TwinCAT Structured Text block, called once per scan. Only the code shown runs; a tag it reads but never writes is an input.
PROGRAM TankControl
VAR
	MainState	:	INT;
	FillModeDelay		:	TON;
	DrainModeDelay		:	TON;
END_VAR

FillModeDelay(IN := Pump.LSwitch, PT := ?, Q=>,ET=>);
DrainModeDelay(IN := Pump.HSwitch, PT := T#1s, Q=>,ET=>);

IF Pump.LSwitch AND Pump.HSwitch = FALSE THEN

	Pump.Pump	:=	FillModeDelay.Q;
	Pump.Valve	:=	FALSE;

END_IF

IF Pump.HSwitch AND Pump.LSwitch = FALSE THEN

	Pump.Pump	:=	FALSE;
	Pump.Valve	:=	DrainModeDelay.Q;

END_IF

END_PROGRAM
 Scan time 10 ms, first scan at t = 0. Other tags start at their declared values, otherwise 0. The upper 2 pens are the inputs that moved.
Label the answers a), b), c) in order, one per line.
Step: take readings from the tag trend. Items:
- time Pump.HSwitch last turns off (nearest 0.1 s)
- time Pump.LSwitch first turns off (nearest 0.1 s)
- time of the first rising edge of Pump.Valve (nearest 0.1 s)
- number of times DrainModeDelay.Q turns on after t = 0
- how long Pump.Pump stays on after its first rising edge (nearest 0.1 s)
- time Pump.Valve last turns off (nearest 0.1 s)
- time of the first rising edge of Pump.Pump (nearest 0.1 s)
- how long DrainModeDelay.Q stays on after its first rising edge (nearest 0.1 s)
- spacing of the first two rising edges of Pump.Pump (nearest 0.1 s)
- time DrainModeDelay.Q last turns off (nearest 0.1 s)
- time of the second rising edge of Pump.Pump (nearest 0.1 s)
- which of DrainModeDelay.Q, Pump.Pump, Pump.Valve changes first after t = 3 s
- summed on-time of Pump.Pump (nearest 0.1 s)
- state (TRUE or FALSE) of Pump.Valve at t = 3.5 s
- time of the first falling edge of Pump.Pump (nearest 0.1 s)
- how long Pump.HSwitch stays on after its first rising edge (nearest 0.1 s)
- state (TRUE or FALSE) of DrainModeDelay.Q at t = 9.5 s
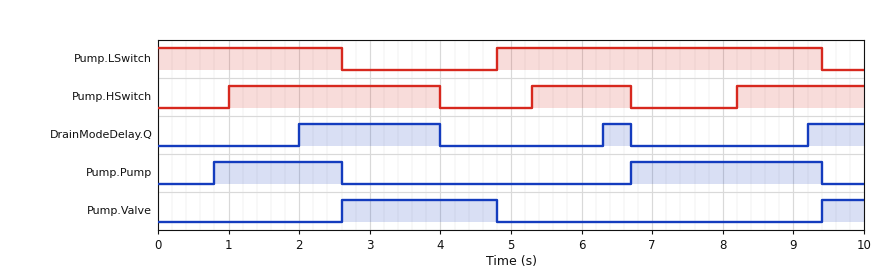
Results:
a) 6.7 s
b) 2.6 s
c) 2.6 s
d) 3
e) 1.8 s
f) 4.8 s
g) 0.8 s
h) 2.0 s
i) 5.9 s
j) 6.7 s
k) 6.7 s
l) DrainModeDelay.Q
m) 4.5 s
n) TRUE
o) 2.6 s
p) 3.0 s
q) TRUE
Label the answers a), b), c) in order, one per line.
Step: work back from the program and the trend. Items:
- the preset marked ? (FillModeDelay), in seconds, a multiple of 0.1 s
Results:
a) 0.8 s
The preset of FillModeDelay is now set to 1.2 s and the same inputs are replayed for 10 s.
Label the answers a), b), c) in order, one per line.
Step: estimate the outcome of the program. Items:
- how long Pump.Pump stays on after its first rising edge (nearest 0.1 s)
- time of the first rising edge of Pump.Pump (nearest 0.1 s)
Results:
a) 2.7 s
b) 6.7 s
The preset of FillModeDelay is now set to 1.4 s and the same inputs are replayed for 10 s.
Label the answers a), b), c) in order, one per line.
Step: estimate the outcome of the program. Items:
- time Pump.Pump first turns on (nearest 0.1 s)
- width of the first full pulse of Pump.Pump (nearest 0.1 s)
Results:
a) 6.7 s
b) 2.7 s
